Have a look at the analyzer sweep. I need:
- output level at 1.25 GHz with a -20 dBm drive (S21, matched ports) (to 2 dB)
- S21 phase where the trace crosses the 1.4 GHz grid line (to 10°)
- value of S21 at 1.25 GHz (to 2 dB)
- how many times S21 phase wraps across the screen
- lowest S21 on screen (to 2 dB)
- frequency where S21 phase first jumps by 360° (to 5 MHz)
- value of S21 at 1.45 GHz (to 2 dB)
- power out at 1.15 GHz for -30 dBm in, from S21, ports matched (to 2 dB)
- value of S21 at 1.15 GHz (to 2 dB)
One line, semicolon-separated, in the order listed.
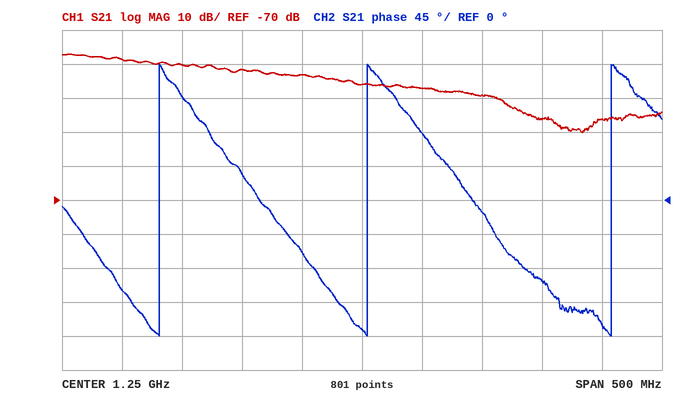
-56 dBm; -110°; -36 dB; 3; -50 dB; 1.080 GHz; -46 dB; -62 dBm; -32 dB
